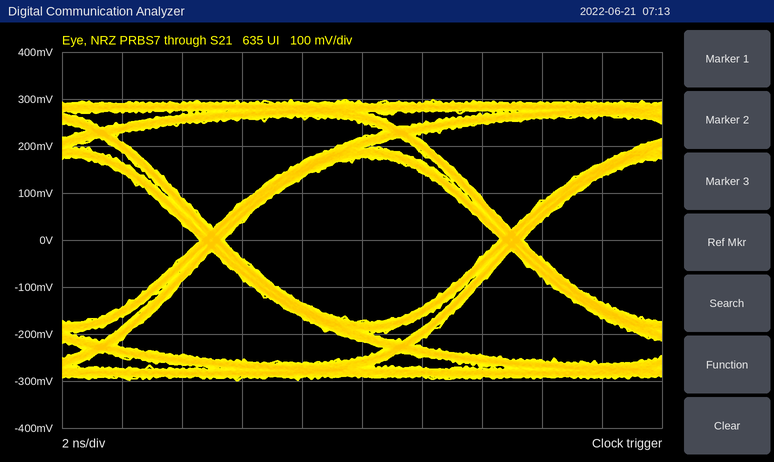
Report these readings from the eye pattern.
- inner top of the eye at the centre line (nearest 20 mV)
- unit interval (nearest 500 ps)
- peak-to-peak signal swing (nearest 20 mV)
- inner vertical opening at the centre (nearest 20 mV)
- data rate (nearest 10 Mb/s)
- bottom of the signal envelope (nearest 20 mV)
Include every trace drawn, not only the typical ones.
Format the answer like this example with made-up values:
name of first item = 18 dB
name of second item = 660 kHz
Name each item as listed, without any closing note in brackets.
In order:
inner top of the eye at the centre line = 180 mV
unit interval = 10.0 ns
peak-to-peak signal swing = 600 mV
inner vertical opening at the centre = 340 mV
data rate = 100 Mb/s
bottom of the signal envelope = -300 mV
